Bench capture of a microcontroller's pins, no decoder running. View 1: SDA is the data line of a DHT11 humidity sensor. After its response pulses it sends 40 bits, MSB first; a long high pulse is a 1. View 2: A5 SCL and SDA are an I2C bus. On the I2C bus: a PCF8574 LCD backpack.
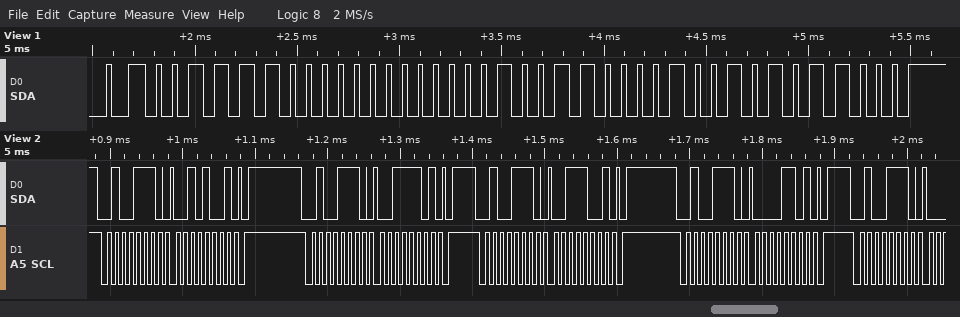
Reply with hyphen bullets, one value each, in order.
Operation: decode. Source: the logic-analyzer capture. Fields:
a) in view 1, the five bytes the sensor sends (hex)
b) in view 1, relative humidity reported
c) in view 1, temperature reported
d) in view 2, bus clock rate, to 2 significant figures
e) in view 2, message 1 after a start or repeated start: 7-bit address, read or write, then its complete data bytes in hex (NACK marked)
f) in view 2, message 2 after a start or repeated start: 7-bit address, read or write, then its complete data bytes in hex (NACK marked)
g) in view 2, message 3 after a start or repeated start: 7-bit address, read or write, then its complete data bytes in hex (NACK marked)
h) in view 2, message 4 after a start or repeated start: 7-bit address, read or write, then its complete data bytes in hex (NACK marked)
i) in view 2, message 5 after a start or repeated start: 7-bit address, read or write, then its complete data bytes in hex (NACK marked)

- 3C 00 13 09 58
- 60 %
- 19.9 °C
- 100 kHz
- 0x27 write: 29
- 0x27 write: 3D
- 0x27 write: 39
- 0x27 write: 0D
- 0x27 write
